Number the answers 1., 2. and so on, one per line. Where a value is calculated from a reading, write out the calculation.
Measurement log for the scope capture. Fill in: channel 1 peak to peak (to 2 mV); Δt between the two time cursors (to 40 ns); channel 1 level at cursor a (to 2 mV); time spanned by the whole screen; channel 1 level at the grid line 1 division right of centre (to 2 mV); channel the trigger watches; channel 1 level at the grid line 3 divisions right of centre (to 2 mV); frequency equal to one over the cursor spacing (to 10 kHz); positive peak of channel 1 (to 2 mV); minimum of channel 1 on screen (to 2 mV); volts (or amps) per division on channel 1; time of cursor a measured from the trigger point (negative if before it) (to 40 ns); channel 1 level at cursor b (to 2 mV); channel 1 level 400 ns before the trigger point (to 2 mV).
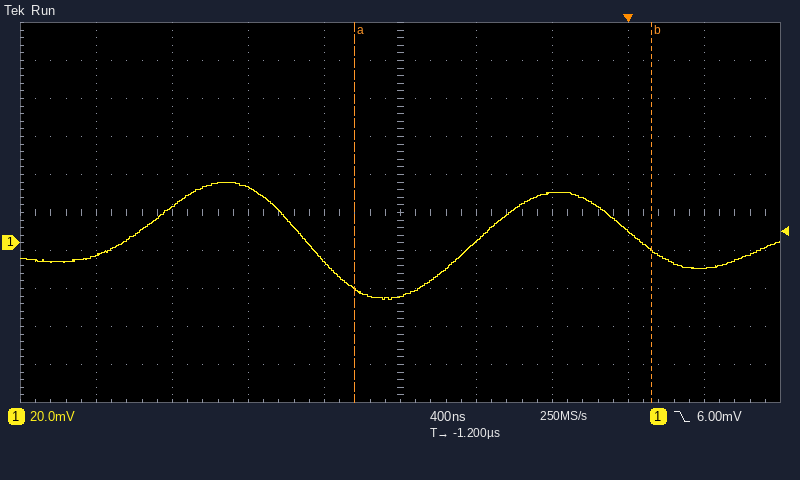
1. 32 mV − (-30 mV) = 62 mV
2. 1.56 µs
3. -24 mV
4. 4 µs
5. 0 mV
6. channel 1
7. 6 mV
8. 1 / 1.56 µs ≈ 640 kHz
9. 32 mV
10. -30 mV
11. 20 mV
12. -1.44 µs
13. -4 mV
14. 26 mV
